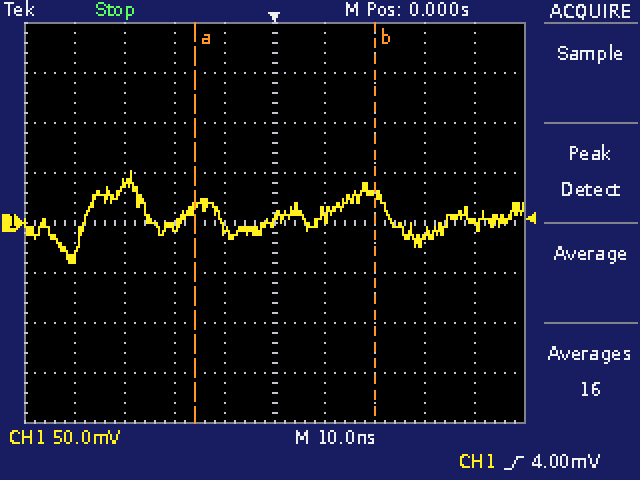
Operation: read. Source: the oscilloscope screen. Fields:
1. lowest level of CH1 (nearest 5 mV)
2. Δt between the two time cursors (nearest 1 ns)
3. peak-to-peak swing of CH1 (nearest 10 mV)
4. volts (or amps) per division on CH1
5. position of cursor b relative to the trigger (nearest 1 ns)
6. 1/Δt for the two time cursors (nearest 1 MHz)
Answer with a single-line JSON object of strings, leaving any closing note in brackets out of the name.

{"lowest level of CH1": "-40 mV", "Δt between the two time cursors": "36 ns", "peak-to-peak swing of CH1": "90 mV", "volts (or amps) per division on CH1": "50 mV", "position of cursor b relative to the trigger": "+20 ns", "1/Δt for the two time cursors": "28 MHz"}
